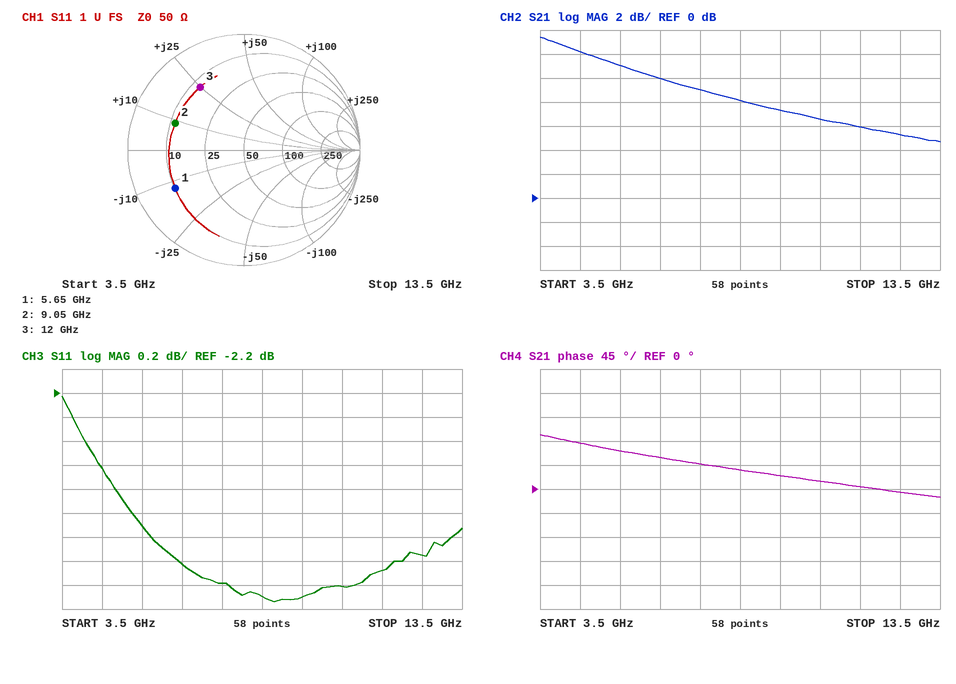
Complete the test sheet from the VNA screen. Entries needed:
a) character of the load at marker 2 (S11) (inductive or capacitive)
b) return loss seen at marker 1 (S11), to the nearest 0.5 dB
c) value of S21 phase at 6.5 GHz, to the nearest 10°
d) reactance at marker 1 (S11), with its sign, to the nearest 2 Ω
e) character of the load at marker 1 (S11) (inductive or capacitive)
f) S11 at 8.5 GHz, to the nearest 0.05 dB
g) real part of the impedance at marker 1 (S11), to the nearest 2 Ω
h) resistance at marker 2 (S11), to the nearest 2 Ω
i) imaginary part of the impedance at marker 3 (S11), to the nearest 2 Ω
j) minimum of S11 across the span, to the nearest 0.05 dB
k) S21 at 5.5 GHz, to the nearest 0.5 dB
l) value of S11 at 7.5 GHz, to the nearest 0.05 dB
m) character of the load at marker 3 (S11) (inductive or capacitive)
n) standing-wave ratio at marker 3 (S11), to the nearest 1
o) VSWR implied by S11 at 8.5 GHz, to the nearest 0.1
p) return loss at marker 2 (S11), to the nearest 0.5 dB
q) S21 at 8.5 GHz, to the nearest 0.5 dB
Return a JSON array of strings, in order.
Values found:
["inductive", "3.5 dB", "60°", "-12 Ω", "capacitive", "-3.90 dB", "10 Ω", "12 Ω", "+24 Ω", "-3.95 dB", "11.0 dB", "-3.80 dB", "inductive", "5", "4.5", "4.0 dB", "8.0 dB"]
